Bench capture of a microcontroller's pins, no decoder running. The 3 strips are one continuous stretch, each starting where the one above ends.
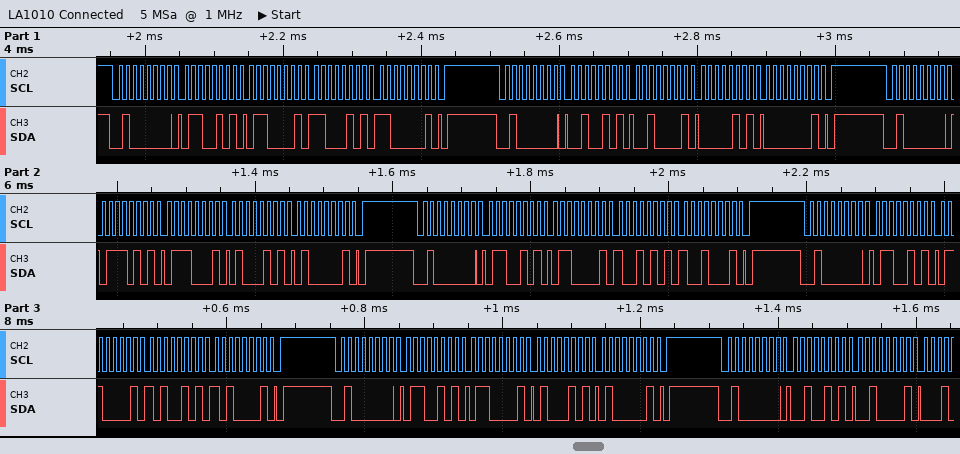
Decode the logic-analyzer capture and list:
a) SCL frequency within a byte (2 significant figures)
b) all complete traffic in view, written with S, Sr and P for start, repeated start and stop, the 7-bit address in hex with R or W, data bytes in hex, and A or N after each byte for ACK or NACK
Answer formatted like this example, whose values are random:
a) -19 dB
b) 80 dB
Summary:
a) 100 kHz
b) S 20W A 65 A 61 A C5 A C1 A P S 20W A 25 A 21 A 05 A 01 A P S 20W A 75 A 71 A 45 A 41 A P S 20W A 65 A 61 A 95 A 91 A P S 20W A 65 A 61 A A5 A A1 A P S 20W A 65 A 61 A 45 A 41 A P S 20W A 25 A 21 A
